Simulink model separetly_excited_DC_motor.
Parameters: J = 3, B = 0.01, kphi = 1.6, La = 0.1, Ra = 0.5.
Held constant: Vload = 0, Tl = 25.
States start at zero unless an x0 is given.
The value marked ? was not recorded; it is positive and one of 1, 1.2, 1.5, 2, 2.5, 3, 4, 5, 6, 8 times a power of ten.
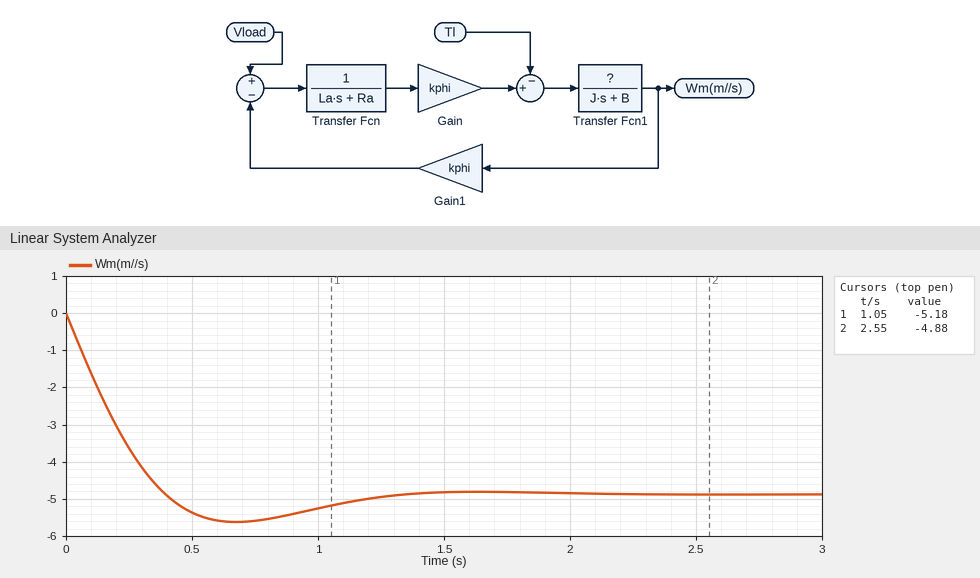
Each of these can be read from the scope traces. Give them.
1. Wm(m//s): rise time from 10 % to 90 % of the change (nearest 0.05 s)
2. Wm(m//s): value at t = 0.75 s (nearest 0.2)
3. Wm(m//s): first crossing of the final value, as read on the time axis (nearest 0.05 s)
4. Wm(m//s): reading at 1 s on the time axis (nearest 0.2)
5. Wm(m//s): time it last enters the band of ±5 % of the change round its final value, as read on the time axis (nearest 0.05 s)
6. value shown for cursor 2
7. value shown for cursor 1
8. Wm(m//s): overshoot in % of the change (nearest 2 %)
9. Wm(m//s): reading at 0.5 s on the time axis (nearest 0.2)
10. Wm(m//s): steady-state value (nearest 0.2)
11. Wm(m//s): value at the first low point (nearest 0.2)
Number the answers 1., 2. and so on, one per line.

1. 0.30 s
2. -5.6
3. 0.40 s
4. -5.2
5. 1.10 s
6. -4.88
7. -5.18
8. 16 %
9. -5.4
10. -4.8
11. -5.6
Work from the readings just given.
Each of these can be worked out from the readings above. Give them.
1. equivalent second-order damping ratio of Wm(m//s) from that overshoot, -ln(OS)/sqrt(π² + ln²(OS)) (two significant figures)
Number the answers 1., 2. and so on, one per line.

1. 0.50
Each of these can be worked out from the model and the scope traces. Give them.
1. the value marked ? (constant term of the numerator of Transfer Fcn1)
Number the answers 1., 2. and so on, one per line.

1. 2
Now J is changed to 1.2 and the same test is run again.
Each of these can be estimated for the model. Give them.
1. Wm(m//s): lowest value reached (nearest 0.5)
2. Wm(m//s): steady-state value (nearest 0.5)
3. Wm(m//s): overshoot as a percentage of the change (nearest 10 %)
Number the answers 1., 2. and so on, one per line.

1. -7.5
2. -5.0
3. 60 %
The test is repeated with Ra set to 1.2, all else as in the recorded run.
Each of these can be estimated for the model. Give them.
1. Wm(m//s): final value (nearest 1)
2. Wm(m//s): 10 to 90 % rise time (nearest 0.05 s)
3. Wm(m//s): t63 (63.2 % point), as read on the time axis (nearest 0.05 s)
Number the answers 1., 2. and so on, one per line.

1. -12
2. 1.35 s
3. 0.60 s
